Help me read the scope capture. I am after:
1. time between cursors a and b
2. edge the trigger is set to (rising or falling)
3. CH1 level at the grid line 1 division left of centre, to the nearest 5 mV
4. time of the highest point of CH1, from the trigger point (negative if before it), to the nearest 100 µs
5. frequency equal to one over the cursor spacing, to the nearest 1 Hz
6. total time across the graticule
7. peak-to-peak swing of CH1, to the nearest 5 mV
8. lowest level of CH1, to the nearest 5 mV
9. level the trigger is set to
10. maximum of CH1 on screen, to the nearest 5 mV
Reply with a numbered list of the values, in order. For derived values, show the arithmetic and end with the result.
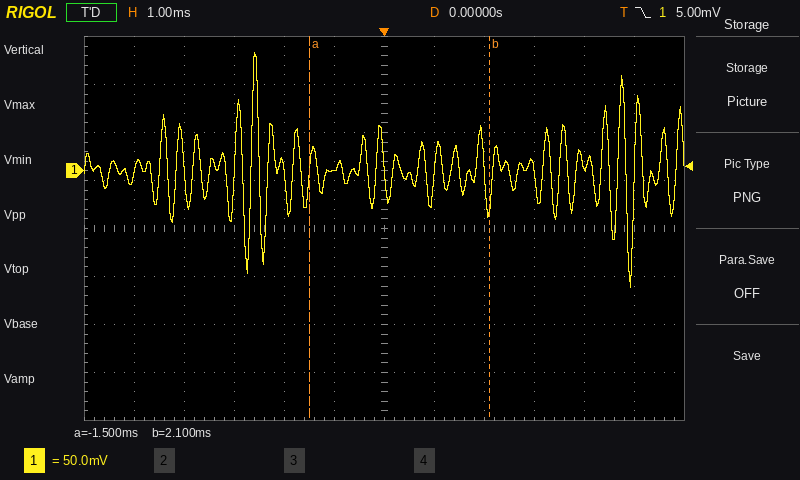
1. 2.1 ms − (-1.5 ms) = 3.6 ms
2. falling
3. 0 mV
4. -2.6 ms
5. 1 / 3.6 ms ≈ 278 Hz
6. 12 ms
7. 125 mV − (-120 mV) = 245 mV
8. -120 mV
9. 5.00 mV
10. 125 mV
